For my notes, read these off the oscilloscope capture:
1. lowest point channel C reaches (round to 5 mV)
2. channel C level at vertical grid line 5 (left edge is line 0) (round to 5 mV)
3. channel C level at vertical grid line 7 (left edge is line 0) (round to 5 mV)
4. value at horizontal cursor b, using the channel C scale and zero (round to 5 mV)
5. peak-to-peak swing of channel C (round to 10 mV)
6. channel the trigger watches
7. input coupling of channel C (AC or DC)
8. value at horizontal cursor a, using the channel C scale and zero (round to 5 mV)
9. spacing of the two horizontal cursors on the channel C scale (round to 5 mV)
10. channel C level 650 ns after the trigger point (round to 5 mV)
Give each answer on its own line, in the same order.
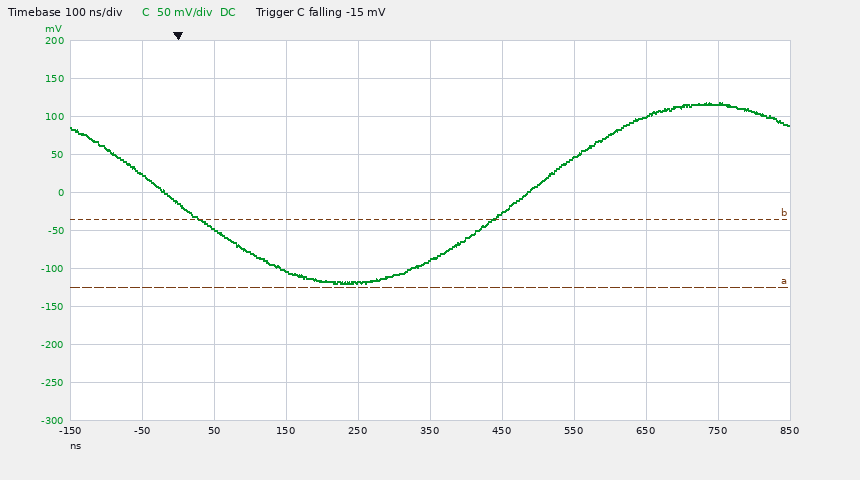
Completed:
-120 mV
-90 mV
45 mV
-35 mV
240 mV
channel C
DC
-125 mV
90 mV
100 mV
